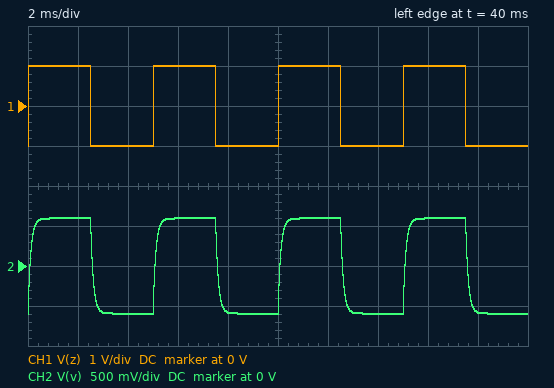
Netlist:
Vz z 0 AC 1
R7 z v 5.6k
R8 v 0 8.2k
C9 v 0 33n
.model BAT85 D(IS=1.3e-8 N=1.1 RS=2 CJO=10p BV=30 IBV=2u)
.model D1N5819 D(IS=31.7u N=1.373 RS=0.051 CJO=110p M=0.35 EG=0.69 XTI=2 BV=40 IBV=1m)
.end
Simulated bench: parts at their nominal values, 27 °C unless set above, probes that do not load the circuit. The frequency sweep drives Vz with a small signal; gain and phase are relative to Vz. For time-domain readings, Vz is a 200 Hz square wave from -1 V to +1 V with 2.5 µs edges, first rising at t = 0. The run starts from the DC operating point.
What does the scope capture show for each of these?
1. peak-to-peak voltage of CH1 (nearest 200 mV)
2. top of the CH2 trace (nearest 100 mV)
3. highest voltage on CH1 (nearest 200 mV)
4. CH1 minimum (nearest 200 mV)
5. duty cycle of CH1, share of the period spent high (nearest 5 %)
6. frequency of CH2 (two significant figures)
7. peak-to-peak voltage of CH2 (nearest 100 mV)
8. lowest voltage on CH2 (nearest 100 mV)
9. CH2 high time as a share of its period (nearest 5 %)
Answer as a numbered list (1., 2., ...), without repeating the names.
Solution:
1. 2.0 V
2. 600 mV
3. 1.0 V
4. -1.0 V
5. 50 %
6. 200 Hz
7. 1.2 V
8. -600 mV
9. 50 %
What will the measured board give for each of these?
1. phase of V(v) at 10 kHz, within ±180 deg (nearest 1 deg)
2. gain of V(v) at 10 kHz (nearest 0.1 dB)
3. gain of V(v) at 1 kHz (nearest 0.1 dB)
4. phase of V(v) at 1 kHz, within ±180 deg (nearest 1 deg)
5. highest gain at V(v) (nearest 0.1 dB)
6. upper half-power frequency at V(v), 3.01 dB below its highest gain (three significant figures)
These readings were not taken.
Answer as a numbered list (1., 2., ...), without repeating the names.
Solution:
1. -82 deg
2. -21.4 dB
3. -6.2 dB
4. -35 deg
5. -4.5 dB
6. 1.45 kHz
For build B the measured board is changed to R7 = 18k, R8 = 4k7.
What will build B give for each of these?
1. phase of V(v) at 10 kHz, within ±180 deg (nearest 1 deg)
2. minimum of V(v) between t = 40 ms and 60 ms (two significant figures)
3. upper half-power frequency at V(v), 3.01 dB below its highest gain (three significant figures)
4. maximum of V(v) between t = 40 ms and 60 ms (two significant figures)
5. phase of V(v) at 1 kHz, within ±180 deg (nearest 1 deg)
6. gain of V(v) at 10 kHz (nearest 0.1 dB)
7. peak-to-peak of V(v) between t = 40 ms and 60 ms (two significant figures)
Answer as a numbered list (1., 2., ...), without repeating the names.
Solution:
1. -83 deg
2. -210 mV
3. 1.29 kHz
4. 210 mV
5. -38 deg
6. -31.5 dB
7. 410 mV
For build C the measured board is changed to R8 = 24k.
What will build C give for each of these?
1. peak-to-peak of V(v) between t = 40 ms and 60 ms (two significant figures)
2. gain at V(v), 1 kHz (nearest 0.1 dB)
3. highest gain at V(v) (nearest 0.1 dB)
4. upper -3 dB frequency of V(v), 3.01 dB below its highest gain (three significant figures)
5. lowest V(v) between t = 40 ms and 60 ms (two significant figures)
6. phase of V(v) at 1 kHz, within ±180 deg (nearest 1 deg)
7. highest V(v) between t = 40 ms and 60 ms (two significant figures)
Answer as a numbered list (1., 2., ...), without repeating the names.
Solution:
1. 1.6 V
2. -4.6 dB
3. -1.8 dB
4. 1.06 kHz
5. -810 mV
6. -43 deg
7. 810 mV
